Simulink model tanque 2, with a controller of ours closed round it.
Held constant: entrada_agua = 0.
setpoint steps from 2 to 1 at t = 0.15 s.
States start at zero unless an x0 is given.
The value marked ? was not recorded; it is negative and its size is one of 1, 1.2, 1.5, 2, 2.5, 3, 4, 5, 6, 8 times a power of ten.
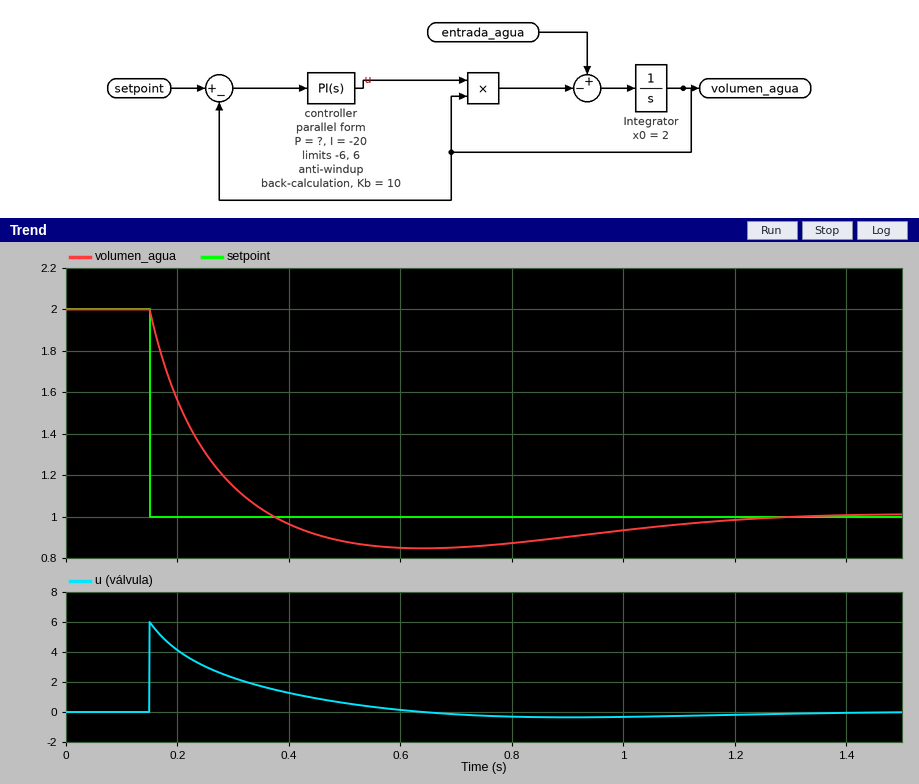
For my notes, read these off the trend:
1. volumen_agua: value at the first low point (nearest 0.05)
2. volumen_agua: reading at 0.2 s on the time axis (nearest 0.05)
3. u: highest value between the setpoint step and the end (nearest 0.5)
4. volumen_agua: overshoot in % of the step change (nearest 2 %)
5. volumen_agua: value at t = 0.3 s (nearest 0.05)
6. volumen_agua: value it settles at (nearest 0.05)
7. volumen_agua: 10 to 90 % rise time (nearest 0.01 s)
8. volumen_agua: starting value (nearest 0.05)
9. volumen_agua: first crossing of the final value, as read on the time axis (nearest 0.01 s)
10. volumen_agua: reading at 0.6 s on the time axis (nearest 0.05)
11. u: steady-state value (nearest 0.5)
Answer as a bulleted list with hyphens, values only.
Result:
- 0.85
- 1.55
- 6.0
- 16 %
- 1.15
- 1.00
- 0.16 s
- 2.00
- 0.37 s
- 0.85
- 0.0
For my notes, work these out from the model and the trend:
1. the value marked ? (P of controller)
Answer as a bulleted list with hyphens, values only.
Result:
- -6
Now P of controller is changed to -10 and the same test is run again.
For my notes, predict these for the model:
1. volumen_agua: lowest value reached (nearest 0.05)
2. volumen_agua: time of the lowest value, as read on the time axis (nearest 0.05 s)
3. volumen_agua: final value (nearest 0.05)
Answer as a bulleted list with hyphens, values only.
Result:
- 0.95
- 0.60 s
- 1.00
